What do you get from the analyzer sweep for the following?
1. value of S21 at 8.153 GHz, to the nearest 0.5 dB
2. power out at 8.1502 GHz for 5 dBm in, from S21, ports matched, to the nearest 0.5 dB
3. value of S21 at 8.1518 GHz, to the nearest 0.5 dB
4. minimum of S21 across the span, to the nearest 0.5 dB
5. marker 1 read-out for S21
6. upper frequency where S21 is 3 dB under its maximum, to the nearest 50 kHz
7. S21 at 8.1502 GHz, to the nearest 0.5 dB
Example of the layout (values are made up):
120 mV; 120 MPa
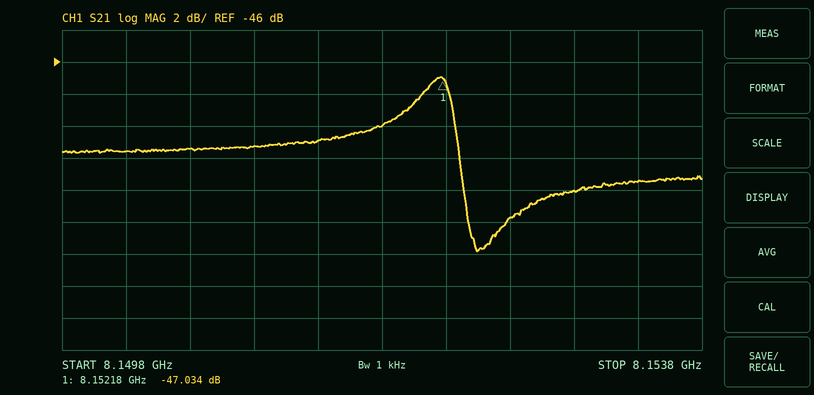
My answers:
-54.0 dB; -46.5 dBm; -50.0 dB; -58.0 dB; -47.034 dB; 8.15225 GHz; -51.5 dB
